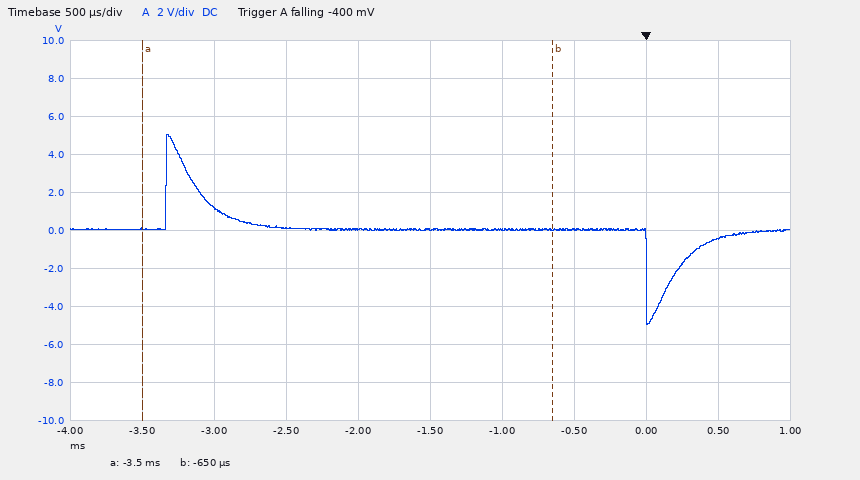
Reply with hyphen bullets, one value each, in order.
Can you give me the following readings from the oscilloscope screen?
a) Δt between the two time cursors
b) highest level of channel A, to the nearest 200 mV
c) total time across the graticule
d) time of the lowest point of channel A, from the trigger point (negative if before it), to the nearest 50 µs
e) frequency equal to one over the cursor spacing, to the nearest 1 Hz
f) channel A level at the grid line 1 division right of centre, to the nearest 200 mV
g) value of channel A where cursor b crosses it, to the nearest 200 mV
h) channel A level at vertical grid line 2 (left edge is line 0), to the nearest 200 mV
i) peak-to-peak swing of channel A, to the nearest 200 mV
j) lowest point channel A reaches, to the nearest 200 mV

- 2.85 ms
- 5.0 V
- 5 ms
- 0 µs
- 351 Hz
- 0.0 V
- 0.0 V
- 1.2 V
- 10.0 V
- -5.0 V
